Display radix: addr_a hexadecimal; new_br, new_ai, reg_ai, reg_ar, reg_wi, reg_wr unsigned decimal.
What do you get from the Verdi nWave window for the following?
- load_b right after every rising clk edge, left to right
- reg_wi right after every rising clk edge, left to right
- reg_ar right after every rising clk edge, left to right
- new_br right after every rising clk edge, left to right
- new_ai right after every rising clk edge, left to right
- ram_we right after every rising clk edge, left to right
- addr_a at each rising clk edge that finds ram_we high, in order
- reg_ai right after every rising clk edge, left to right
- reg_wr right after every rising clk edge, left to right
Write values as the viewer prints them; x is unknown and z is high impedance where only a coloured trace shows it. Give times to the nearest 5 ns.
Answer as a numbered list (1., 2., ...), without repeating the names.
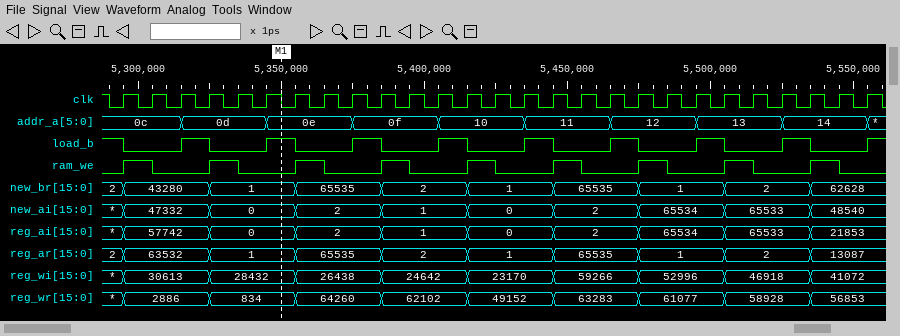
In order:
1. 0 0 1 0 0 1 0 0 1 0 0 1 0 0 1 0 0 1 0 0 1 0 0 1 0 0 1
2. 30613, 30613, 30613, 28432, 28432, 28432, 26438, 26438, 26438, 24642, 24642, 24642, 23170, 23170, 23170, 59266, 59266, 59266, 52996, 52996, 52996, 46918, 46918, 46918, 41072, 41072, 41072
3. 63532, 63532, 63532, 1, 1, 1, 65535, 65535, 65535, 2, 2, 2, 1, 1, 1, 65535, 65535, 65535, 1, 1, 1, 2, 2, 2, 13087, 13087, 13087
4. 43280, 43280, 43280, 1, 1, 1, 65535, 65535, 65535, 2, 2, 2, 1, 1, 1, 65535, 65535, 65535, 1, 1, 1, 2, 2, 2, 62628, 62628, 62628
5. 47332, 47332, 47332, 0, 0, 0, 2, 2, 2, 1, 1, 1, 0, 0, 0, 2, 2, 2, 65534, 65534, 65534, 65533, 65533, 65533, 48540, 48540, 48540
6. 1 0 0 1 0 0 1 0 0 1 0 0 1 0 0 1 0 0 1 0 0 1 0 0 1 0 0
7. 0c, 0d, 0e, 0f, 10, 11, 12, 13, 14
8. 57742, 57742, 57742, 0, 0, 0, 2, 2, 2, 1, 1, 1, 0, 0, 0, 2, 2, 2, 65534, 65534, 65534, 65533, 65533, 65533, 21853, 21853, 21853
9. 2886, 2886, 2886, 834, 834, 834, 64260, 64260, 64260, 62102, 62102, 62102, 49152, 49152, 49152, 63283, 63283, 63283, 61077, 61077, 61077, 58928, 58928, 58928, 56853, 56853, 56853
